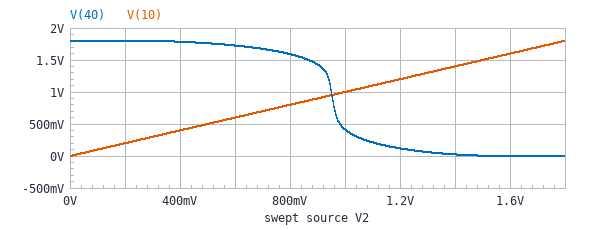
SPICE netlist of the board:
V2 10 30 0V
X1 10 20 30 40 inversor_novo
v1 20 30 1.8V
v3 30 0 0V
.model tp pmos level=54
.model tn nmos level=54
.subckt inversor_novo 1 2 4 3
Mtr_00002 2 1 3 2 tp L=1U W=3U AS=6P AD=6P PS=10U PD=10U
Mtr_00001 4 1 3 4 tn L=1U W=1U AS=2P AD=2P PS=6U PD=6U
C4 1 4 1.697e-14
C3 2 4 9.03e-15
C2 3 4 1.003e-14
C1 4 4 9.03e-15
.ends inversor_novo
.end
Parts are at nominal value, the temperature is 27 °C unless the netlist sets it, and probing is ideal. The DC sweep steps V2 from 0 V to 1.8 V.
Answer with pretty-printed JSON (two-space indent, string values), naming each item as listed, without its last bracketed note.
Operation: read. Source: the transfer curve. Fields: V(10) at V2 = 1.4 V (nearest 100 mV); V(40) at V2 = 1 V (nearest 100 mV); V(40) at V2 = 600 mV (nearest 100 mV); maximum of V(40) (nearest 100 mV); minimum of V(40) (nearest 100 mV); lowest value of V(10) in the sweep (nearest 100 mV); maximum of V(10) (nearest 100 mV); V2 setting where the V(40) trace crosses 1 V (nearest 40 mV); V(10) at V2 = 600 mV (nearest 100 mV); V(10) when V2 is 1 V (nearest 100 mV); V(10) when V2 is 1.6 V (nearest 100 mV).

{
  "V(10) at V2 = 1.4 V": "1.4 V",
  "V(40) at V2 = 1 V": "400 mV",
  "V(40) at V2 = 600 mV": "1.7 V",
  "maximum of V(40)": "1.8 V",
  "minimum of V(40)": "0 V",
  "lowest value of V(10) in the sweep": "0 V",
  "maximum of V(10)": "1.8 V",
  "V2 setting where the V(40) trace crosses 1 V": "960 mV",
  "V(10) at V2 = 600 mV": "600 mV",
  "V(10) when V2 is 1 V": "1.0 V",
  "V(10) when V2 is 1.6 V": "1.6 V"
}
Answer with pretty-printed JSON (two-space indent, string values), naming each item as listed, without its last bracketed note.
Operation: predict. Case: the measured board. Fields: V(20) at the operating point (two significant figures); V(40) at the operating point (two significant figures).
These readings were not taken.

{
  "V(20) at the operating point": "1.8 V",
  "V(40) at the operating point": "1.8 V"
}
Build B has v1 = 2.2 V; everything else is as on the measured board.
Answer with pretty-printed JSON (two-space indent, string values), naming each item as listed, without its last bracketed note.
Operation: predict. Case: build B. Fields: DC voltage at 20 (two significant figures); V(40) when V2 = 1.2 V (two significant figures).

{
  "DC voltage at 20": "2.2 V",
  "V(40) when V2 = 1.2 V": "700 mV"
}
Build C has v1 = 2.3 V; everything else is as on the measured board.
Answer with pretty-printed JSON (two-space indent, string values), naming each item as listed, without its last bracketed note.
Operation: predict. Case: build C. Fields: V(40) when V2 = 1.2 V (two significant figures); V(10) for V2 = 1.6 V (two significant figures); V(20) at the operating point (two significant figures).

{
  "V(40) when V2 = 1.2 V": "1.6 V",
  "V(10) for V2 = 1.6 V": "1.6 V",
  "V(20) at the operating point": "2.3 V"
}
